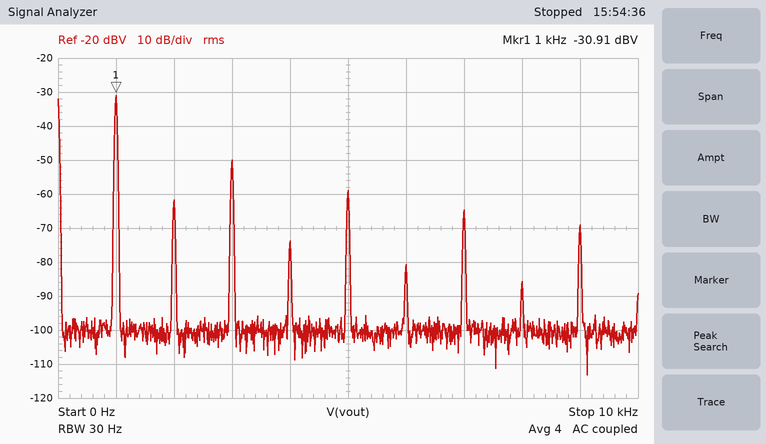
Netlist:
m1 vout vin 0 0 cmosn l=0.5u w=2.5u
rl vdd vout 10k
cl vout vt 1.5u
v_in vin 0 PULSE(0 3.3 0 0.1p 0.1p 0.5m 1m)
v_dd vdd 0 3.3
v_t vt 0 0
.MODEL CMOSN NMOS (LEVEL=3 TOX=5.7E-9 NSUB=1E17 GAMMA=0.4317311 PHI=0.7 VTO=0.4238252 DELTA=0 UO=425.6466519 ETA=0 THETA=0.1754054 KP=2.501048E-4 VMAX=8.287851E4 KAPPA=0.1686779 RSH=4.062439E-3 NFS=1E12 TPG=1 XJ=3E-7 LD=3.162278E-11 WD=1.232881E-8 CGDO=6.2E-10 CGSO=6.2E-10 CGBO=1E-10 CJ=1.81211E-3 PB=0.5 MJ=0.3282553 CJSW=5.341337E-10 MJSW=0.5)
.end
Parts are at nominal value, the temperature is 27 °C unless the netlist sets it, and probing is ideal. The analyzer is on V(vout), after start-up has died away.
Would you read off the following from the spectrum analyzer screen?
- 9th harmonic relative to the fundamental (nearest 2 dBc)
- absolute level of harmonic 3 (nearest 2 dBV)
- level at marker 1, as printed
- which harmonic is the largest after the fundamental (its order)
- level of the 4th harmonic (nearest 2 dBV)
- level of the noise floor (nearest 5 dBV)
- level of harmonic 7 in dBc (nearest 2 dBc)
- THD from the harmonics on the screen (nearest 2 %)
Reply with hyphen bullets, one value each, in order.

- -38 dBc
- -50 dBV
- -30.91 dBV
- 3
- -74 dBV
- -100 dBV
- -34 dBc
- 12 %
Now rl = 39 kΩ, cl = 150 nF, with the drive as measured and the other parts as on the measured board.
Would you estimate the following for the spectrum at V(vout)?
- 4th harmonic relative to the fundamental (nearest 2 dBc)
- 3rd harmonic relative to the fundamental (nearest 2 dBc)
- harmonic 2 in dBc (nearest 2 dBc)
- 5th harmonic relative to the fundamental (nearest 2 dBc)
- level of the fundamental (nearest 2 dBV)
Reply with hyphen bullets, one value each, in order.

- -22 dBc
- -14 dBc
- -12 dBc
- -22 dBc
- -22 dBV
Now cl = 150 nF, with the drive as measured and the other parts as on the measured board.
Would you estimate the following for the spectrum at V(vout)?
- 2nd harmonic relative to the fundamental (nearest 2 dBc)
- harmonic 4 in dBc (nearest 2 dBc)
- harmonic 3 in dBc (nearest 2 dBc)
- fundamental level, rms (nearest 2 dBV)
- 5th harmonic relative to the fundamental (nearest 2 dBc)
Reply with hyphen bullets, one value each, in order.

- -14 dBc
- -26 dBc
- -16 dBc
- -12 dBV
- -26 dBc
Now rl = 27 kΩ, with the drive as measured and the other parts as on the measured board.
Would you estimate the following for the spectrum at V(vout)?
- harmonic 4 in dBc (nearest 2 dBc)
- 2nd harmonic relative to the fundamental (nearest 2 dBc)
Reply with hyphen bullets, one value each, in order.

- -40 dBc
- -28 dBc
